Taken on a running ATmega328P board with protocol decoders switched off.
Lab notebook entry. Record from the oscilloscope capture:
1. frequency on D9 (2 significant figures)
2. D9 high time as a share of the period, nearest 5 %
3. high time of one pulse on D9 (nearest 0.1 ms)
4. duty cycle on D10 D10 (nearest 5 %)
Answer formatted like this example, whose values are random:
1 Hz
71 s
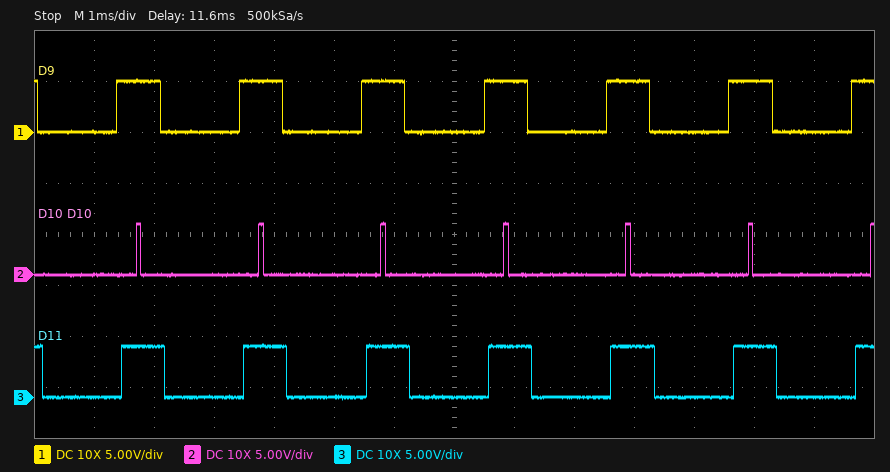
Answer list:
490 Hz
35 %
0.7 ms
5 %
